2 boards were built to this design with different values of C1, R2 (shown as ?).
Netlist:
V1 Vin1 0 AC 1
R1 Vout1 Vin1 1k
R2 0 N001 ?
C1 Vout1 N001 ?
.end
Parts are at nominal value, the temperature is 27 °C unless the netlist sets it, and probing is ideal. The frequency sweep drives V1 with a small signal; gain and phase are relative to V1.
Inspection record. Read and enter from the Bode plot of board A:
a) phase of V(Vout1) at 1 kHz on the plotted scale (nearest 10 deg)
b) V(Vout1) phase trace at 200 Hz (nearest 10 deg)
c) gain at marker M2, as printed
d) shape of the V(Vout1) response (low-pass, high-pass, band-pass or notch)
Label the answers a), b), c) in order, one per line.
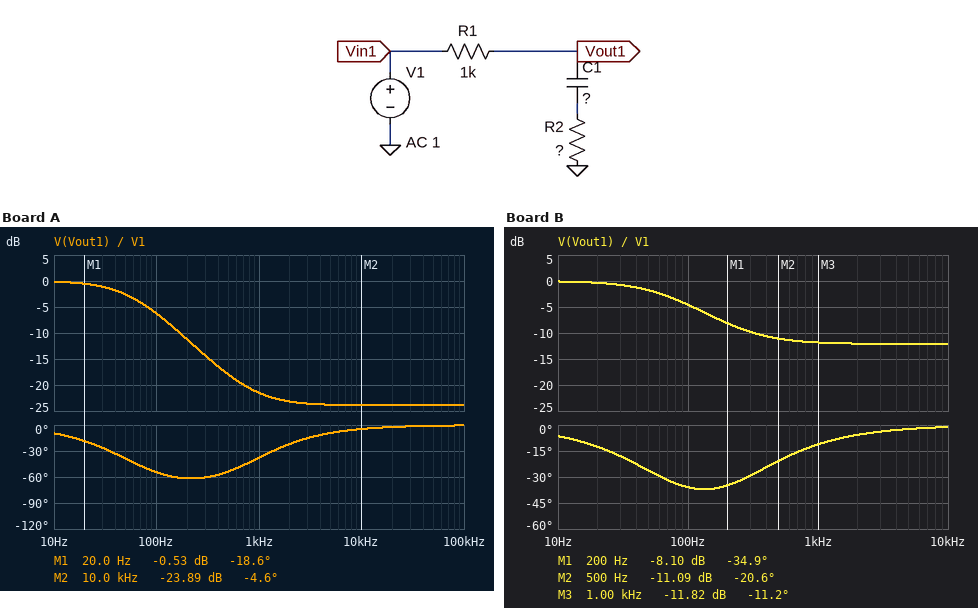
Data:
a) -40 deg
b) -60 deg
c) -23.89 dB
d) low-pass
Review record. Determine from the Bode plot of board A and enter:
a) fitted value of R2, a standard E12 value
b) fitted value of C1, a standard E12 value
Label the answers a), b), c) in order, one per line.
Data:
a) 68 Ω
b) 2.7 µF
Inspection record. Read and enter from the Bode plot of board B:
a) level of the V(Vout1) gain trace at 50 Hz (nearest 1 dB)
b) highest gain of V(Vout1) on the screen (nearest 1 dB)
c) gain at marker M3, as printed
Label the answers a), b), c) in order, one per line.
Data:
a) -2 dB
b) 0 dB
c) -11.82 dB
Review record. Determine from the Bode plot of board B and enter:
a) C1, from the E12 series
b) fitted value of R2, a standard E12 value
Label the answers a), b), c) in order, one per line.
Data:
a) 1.8 µF
b) 330 Ω
